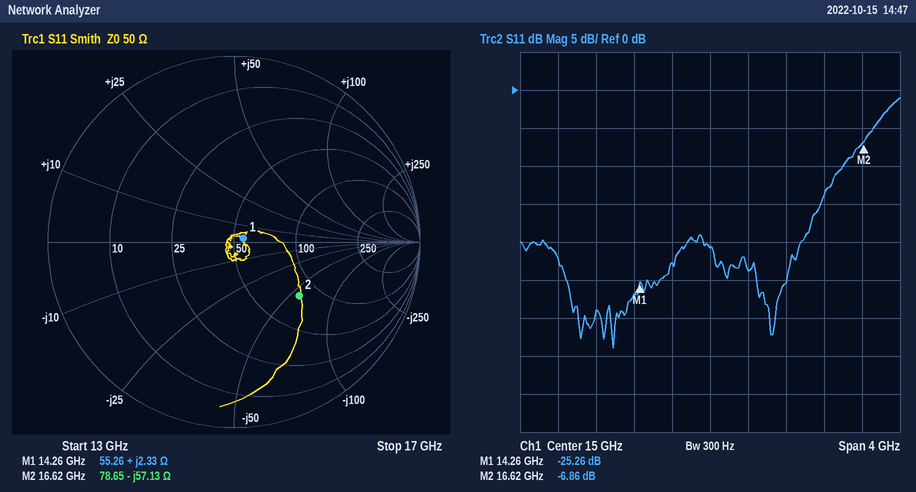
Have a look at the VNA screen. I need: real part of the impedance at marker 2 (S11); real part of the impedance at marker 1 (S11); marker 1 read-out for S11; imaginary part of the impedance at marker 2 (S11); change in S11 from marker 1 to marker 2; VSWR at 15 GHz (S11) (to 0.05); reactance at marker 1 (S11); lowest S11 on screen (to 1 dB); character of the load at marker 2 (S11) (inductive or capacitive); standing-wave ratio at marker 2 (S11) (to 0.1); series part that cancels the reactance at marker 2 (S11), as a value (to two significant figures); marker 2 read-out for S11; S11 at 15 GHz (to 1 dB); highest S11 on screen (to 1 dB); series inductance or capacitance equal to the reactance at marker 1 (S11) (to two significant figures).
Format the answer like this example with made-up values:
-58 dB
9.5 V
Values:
78.65 Ω
55.26 Ω
-25.26 dB
-57.13 Ω
18.40 dB
1.20
+2.33 Ω
-34 dB
capacitive
2.7
550 pH
-6.86 dB
-21 dB
-1 dB
26 pH
